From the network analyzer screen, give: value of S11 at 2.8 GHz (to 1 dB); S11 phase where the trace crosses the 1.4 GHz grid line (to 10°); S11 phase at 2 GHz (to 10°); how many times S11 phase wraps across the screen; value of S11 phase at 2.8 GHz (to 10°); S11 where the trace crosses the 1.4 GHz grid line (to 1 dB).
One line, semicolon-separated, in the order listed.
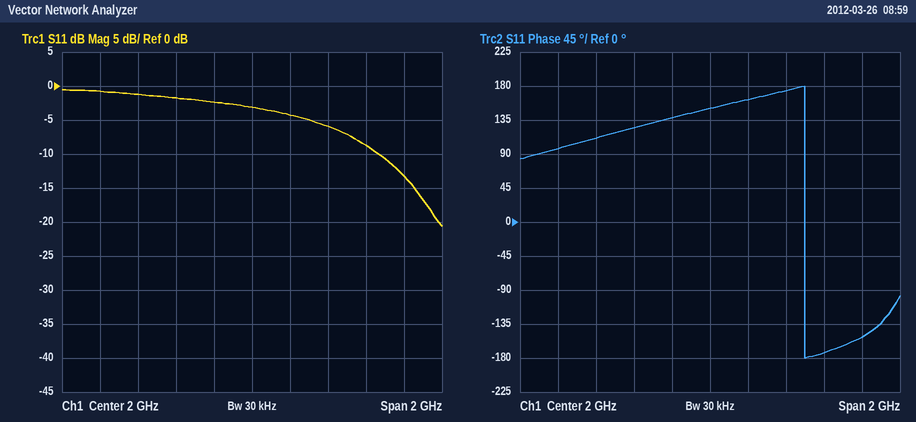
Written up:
-13 dB; 110°; 150°; 1; -150°; -1 dB
